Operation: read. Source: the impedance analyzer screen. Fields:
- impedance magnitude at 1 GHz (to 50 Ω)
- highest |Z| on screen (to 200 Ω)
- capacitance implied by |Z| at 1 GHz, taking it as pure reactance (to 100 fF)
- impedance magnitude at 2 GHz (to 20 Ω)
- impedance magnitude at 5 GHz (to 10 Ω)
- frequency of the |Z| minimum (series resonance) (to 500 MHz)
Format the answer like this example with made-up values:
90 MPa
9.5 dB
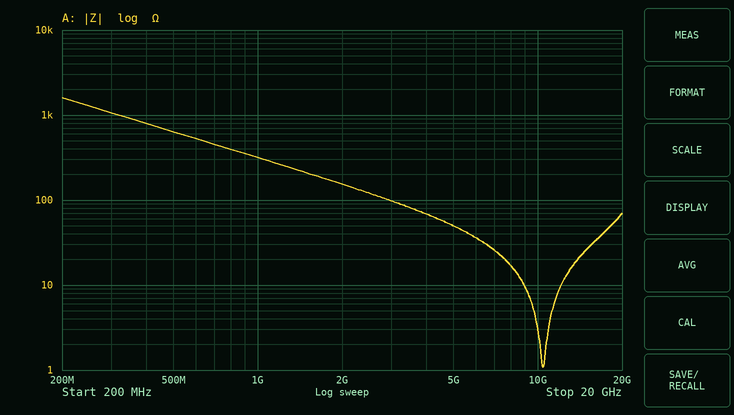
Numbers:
300 Ω
1.6 kΩ
500 fF
160 Ω
50 Ω
10.5 GHz
